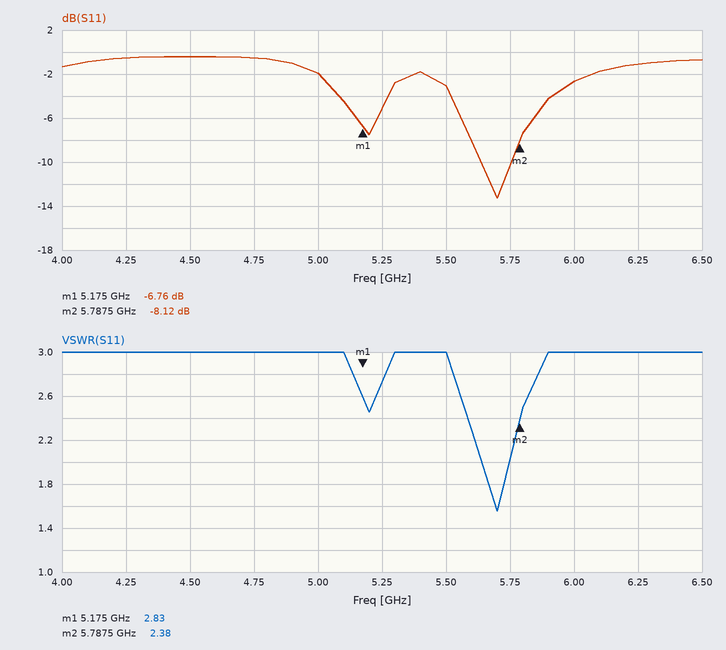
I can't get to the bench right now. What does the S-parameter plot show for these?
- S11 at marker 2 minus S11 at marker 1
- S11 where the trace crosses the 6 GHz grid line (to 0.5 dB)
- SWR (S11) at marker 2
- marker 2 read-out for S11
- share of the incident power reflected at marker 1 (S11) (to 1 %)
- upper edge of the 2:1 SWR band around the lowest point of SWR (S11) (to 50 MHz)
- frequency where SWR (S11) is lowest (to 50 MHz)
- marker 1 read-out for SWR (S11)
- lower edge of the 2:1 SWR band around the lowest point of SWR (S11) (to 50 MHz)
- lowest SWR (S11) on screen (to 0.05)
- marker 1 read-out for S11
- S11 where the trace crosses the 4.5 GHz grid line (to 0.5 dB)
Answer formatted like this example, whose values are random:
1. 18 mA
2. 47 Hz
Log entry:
1. -1.36 dB
2. -2.5 dB
3. 2.38
4. -8.12 dB
5. 21 %
6. 5.75 GHz
7. 5.70 GHz
8. 2.83
9. 5.65 GHz
10. 1.55
11. -6.76 dB
12. -0.5 dB
